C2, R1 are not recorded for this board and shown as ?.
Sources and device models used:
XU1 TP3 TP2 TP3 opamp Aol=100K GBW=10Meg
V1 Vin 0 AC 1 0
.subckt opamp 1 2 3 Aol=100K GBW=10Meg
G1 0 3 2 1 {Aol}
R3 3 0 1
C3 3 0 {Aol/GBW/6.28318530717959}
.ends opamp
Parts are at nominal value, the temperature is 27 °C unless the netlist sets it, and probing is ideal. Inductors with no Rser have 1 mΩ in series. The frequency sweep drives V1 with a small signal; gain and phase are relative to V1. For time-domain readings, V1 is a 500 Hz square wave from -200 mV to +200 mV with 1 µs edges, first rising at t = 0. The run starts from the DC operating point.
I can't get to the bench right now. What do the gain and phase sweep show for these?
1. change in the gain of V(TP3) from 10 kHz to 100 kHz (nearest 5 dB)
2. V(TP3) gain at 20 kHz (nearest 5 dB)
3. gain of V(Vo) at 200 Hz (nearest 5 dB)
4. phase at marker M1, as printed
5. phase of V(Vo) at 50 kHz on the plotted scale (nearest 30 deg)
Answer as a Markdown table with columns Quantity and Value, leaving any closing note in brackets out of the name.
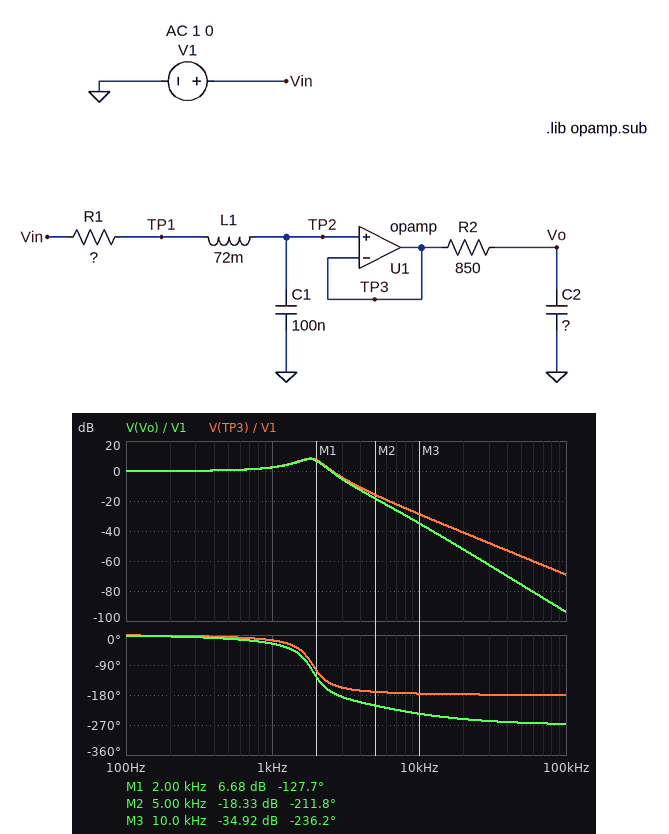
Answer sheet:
| Quantity | Value |
|---|---|
| change in the gain of V(TP3) from 10 kHz to 100 kHz | -40 dB |
| V(TP3) gain at 20 kHz | -40 dB |
| gain of V(Vo) at 200 Hz | 0 dB |
| phase at marker M1, as printed | -127.7 deg |
| phase of V(Vo) at 50 kHz on the plotted scale | -270 deg |
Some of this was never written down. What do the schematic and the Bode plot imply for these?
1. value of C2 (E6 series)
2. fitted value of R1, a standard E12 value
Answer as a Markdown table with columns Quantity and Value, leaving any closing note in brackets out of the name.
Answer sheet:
| Quantity | Value |
|---|---|
| value of C2 | 33 nF |
| fitted value of R1, a standard E12 value | 330 Ω |
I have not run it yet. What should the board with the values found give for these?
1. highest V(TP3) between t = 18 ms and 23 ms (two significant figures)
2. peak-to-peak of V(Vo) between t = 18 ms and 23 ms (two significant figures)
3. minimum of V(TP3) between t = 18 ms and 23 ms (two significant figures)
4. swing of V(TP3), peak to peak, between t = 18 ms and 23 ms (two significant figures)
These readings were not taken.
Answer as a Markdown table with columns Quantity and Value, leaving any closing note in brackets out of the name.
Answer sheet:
| Quantity | Value |
|---|---|
| highest V(TP3) between t = 18 ms and 23 ms | 410 mV |
| peak-to-peak of V(Vo) between t = 18 ms and 23 ms | 790 mV |
| minimum of V(TP3) between t = 18 ms and 23 ms | -410 mV |
| swing of V(TP3), peak to peak, between t = 18 ms and 23 ms | 810 mV |
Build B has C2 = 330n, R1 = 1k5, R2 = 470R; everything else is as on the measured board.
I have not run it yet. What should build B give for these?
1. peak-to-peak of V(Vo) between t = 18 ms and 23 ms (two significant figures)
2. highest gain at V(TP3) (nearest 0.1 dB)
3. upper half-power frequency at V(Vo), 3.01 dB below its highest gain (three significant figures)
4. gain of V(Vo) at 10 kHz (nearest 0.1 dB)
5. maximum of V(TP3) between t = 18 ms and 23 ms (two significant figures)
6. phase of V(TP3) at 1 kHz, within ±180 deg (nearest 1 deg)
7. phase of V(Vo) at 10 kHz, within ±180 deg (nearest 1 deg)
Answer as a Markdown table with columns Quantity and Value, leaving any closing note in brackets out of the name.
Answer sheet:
| Quantity | Value |
|---|---|
| peak-to-peak of V(Vo) between t = 18 ms and 23 ms | 400 mV |
| highest gain at V(TP3) | 0 dB |
| upper half-power frequency at V(Vo), 3.01 dB below its highest gain | 803 Hz |
| gain of V(Vo) at 10 kHz | -49.1 dB |
| maximum of V(TP3) between t = 18 ms and 23 ms | 200 mV |
| phase of V(TP3) at 1 kHz, within ±180 deg | -53 deg |
| phase of V(Vo) at 10 kHz, within ±180 deg | 115 deg |
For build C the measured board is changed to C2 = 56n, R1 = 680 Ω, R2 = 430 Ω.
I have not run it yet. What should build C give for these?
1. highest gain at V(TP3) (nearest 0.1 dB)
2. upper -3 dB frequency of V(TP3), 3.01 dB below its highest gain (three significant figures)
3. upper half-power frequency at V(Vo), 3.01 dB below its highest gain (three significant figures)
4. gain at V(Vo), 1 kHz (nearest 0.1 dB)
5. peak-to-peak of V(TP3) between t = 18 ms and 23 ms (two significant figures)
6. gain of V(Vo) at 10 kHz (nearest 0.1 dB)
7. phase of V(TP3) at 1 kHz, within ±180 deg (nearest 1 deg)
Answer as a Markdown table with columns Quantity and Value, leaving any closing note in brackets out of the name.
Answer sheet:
| Quantity | Value |
|---|---|
| highest gain at V(TP3) | 2.7 dB |
| upper -3 dB frequency of V(TP3), 3.01 dB below its highest gain | 2.23 kHz |
| upper half-power frequency at V(Vo), 3.01 dB below its highest gain | 2.20 kHz |
| gain at V(Vo), 1 kHz | 1.5 dB |
| peak-to-peak of V(TP3) between t = 18 ms and 23 ms | 600 mV |
| gain of V(Vo) at 10 kHz | -34.0 dB |
| phase of V(TP3) at 1 kHz, within ±180 deg | -31 deg |
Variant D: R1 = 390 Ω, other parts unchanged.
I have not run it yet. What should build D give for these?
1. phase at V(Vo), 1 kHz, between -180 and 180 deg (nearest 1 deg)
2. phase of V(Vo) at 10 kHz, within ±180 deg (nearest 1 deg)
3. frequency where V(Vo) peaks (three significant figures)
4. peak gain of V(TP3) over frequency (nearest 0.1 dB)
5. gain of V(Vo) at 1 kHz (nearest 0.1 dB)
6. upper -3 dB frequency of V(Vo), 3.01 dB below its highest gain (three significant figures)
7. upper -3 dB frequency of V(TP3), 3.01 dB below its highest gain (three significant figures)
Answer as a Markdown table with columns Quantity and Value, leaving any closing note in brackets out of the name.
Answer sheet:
| Quantity | Value |
|---|---|
| phase at V(Vo), 1 kHz, between -180 and 180 deg | -29 deg |
| phase of V(Vo) at 10 kHz, within ±180 deg | 125 deg |
| frequency where V(Vo) peaks | 1.76 kHz |
| peak gain of V(TP3) over frequency | 7.0 dB |
| gain of V(Vo) at 1 kHz | 2.3 dB |
| upper -3 dB frequency of V(Vo), 3.01 dB below its highest gain | 2.16 kHz |
| upper -3 dB frequency of V(TP3), 3.01 dB below its highest gain | 2.17 kHz |
